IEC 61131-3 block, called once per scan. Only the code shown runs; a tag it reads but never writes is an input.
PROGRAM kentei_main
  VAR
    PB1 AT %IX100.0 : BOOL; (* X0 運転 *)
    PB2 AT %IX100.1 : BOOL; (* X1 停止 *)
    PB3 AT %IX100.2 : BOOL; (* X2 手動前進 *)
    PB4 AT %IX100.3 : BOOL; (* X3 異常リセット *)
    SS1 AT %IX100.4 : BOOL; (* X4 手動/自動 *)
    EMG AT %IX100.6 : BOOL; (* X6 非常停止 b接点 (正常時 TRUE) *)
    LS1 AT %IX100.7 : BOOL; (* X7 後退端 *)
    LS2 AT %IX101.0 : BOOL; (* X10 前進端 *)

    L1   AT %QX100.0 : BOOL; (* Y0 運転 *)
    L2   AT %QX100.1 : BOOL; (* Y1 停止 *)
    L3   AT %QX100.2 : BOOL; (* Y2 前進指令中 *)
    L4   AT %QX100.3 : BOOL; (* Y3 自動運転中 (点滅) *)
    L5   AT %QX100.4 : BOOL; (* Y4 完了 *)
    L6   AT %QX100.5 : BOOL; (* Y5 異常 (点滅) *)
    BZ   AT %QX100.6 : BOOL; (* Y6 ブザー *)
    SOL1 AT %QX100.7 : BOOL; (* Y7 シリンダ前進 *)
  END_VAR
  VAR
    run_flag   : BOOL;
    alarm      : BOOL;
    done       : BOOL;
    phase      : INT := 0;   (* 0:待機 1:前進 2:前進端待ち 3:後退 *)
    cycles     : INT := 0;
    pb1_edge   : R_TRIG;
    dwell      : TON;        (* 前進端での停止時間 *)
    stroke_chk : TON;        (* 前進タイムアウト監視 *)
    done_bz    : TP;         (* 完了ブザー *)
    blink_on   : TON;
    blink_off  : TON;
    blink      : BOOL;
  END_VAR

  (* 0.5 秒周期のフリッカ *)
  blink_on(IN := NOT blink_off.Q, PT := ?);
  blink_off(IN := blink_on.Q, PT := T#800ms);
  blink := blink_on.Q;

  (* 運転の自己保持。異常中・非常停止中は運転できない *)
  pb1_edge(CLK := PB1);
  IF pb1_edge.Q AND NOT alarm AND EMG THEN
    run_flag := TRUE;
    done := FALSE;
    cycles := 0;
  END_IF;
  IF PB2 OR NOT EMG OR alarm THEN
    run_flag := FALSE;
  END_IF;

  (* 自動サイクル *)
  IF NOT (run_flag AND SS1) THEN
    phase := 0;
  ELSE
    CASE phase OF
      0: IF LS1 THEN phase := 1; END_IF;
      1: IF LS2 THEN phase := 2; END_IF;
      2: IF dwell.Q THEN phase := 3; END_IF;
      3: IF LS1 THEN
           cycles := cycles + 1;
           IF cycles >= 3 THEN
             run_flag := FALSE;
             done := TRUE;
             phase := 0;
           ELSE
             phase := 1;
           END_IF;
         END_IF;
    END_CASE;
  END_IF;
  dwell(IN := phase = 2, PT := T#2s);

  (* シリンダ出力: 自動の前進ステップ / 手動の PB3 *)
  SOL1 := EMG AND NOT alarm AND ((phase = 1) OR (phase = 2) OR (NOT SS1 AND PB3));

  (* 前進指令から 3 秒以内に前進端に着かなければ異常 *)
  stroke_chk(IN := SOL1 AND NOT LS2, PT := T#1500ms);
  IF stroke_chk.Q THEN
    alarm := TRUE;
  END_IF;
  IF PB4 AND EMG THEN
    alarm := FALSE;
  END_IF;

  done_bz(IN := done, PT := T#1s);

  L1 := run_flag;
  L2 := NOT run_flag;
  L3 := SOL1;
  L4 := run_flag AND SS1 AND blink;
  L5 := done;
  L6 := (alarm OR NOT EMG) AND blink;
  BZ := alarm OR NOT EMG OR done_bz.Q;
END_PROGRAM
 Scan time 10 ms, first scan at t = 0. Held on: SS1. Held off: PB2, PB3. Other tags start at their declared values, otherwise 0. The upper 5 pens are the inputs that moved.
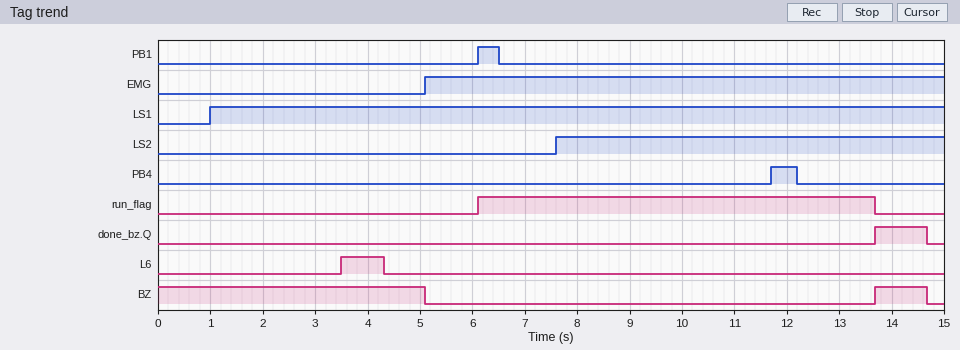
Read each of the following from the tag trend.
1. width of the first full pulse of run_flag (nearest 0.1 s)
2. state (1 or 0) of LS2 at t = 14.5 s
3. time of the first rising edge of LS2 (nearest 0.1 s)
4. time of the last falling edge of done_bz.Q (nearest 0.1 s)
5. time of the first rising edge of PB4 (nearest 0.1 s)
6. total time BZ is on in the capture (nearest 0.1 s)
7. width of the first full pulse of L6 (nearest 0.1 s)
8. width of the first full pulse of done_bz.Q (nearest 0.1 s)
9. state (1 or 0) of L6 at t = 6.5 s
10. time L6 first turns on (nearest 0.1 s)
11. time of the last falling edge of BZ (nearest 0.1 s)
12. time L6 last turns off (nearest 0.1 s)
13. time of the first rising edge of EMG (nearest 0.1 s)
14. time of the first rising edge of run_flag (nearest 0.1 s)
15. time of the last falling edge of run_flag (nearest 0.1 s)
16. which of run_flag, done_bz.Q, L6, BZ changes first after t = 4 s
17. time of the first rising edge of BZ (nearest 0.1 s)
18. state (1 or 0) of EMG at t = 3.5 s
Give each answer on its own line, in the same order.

7.6 s
1
7.6 s
14.7 s
11.7 s
6.1 s
0.8 s
1.0 s
0
3.5 s
14.7 s
4.3 s
5.1 s
6.1 s
13.7 s
L6
13.7 s
0
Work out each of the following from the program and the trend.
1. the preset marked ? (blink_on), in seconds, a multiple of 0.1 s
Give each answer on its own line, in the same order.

3.5 s
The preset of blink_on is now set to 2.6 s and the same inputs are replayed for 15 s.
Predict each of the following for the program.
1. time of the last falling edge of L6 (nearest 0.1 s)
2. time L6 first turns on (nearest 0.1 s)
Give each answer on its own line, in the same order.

3.4 s
2.6 s
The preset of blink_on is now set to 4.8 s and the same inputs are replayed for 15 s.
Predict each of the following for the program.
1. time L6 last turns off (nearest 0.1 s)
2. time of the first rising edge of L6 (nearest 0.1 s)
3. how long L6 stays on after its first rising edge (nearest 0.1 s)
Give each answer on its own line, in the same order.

5.1 s
4.8 s
0.3 s
